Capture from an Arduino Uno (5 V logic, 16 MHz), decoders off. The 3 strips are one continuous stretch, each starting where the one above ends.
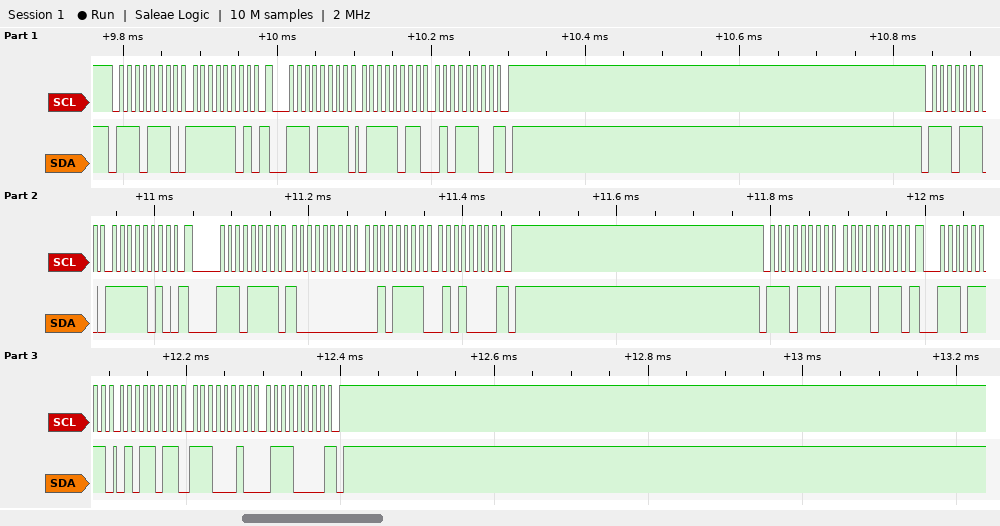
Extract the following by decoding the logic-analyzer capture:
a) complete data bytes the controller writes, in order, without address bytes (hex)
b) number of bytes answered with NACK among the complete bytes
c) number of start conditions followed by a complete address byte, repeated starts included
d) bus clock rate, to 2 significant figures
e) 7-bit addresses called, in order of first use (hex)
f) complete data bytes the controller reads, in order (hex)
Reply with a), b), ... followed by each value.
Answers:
a) FD FA F7
b) 3
c) 6
d) 100 kHz
e) 0x77
f) 7B 5C 80 2F 50 5B E2 70
